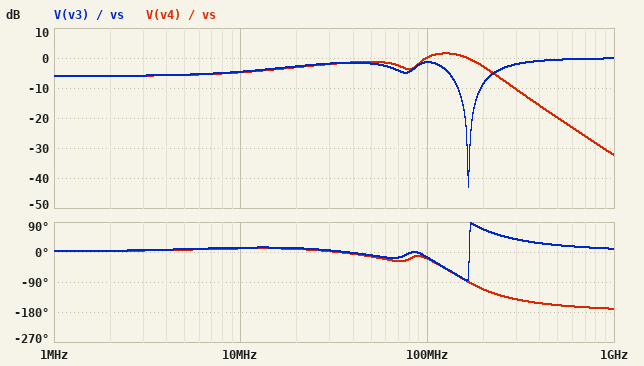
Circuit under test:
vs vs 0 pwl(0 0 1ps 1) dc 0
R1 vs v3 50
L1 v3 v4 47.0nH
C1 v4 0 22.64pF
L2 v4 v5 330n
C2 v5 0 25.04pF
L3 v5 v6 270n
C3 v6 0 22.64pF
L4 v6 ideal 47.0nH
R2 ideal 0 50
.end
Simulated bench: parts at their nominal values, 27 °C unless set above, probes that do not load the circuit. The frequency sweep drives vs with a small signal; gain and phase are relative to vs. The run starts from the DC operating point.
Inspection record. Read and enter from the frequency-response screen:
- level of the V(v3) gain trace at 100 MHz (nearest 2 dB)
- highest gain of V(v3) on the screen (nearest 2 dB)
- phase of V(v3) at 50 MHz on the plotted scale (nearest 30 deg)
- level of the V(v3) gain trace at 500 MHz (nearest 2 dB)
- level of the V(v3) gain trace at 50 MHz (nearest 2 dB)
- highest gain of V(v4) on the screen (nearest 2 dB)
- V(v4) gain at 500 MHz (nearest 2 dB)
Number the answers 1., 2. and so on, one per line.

1. -2 dB
2. 0 dB
3. 0 deg
4. 0 dB
5. -2 dB
6. 2 dB
7. -20 dB
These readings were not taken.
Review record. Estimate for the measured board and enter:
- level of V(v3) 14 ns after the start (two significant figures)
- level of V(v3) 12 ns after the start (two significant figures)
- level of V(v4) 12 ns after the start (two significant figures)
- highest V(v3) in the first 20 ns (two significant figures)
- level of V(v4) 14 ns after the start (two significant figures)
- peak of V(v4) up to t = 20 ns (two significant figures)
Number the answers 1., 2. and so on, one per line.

1. 580 mV
2. 660 mV
3. 630 mV
4. 1.0 V
5. 540 mV
6. 920 mV
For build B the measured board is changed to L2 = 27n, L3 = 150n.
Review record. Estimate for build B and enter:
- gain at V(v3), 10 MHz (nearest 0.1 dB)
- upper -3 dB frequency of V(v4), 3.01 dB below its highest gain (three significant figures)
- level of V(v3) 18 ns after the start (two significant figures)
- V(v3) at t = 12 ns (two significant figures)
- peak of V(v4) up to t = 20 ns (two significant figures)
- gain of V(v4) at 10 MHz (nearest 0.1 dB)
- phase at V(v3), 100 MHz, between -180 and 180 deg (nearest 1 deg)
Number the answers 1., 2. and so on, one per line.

1. -5.8 dB
2. 315 MHz
3. 520 mV
4. 530 mV
5. 770 mV
6. -5.9 dB
7. -24 deg
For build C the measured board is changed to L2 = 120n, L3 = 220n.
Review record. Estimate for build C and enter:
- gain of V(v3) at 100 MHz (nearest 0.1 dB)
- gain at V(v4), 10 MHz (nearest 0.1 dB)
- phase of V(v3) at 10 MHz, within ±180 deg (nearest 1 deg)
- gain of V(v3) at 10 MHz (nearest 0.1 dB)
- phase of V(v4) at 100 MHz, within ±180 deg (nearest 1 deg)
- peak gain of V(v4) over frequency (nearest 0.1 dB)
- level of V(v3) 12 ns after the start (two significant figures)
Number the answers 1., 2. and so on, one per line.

1. -11.0 dB
2. -5.5 dB
3. 8 deg
4. -5.4 dB
5. -57 deg
6. 2.6 dB
7. 460 mV
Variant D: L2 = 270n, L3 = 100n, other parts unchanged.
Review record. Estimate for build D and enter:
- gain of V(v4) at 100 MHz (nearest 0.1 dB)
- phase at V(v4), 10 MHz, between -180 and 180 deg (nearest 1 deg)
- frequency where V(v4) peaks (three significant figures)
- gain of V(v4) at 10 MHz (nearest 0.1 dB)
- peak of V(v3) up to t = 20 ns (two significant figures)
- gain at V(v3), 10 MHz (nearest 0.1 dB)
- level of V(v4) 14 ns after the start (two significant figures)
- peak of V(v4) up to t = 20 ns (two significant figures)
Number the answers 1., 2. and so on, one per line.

1. -0.3 dB
2. 6 deg
3. 135 MHz
4. -5.5 dB
5. 1.0 V
6. -5.4 dB
7. 510 mV
8. 890 mV
